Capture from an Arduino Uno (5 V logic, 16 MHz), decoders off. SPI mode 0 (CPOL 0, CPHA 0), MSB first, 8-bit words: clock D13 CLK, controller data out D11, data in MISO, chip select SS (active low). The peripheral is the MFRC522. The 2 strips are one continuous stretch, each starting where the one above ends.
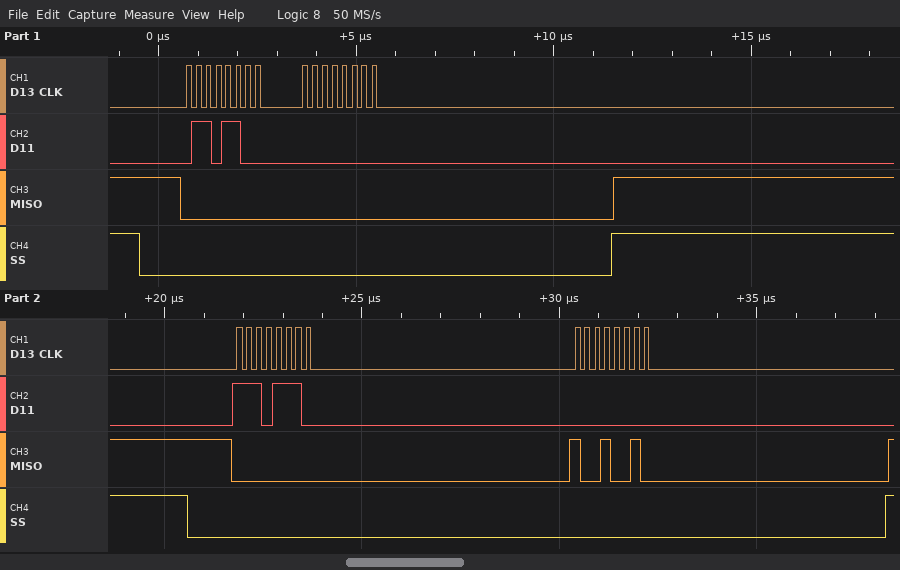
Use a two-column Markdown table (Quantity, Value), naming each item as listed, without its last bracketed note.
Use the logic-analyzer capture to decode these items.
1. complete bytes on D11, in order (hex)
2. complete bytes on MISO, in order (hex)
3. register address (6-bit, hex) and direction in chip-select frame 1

| Quantity | Value |
|---|---|
| complete bytes on D11, in order | 6C 00 EE 00 |
| complete bytes on MISO, in order | 00 00 00 92 |
| register address (6-bit, hex) and direction in chip-select frame 1 | 0x36 write |
